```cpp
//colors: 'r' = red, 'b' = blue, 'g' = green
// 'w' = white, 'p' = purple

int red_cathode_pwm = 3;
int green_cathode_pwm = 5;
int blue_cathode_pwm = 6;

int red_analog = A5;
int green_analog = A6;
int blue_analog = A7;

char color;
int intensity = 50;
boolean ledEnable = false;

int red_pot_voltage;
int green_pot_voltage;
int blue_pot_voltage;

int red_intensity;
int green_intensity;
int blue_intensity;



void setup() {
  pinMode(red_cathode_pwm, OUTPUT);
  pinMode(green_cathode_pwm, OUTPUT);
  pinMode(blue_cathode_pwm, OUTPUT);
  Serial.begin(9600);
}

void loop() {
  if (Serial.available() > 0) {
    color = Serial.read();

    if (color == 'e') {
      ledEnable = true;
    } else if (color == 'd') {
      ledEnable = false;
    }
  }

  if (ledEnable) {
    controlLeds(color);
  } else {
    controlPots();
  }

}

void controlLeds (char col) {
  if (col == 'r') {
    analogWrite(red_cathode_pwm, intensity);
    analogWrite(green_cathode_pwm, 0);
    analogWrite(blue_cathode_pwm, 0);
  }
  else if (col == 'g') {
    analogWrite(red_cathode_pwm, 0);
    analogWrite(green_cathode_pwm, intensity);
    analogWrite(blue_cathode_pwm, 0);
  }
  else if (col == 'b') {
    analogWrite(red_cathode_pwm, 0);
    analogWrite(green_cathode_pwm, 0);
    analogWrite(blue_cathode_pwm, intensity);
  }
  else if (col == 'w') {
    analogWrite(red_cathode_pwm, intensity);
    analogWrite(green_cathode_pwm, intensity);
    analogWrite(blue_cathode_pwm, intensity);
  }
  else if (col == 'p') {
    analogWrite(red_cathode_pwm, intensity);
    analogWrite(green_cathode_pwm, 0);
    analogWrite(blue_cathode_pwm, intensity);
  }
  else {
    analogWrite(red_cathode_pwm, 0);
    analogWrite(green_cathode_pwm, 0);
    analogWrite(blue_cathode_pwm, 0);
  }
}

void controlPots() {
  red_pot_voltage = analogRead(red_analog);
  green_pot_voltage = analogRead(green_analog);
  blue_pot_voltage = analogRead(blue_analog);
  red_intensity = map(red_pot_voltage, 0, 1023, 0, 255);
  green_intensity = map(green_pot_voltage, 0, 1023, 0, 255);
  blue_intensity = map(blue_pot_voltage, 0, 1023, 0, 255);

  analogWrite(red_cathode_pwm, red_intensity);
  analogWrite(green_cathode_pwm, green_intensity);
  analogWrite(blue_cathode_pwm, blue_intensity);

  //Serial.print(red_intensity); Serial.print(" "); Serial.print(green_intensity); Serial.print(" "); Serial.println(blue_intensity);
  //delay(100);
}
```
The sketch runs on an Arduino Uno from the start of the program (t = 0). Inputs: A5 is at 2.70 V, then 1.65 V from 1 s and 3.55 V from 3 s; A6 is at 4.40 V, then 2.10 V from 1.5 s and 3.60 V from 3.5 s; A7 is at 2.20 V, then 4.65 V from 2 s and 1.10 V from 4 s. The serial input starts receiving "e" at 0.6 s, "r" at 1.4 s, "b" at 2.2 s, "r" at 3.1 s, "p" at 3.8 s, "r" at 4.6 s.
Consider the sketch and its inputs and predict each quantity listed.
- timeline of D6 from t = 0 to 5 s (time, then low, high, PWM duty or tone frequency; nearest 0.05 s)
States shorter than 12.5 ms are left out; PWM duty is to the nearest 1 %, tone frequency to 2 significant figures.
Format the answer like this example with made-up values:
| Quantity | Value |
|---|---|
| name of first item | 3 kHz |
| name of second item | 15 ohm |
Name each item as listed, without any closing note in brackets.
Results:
| Quantity | Value |
|---|---|
| timeline of D6 from t = 0 to 5 s | 0 s PWM 44 %; 0.6 s low; 2.2 s PWM 20 %; 3.1 s low; 3.8 s PWM 20 %; 4.6 s low |
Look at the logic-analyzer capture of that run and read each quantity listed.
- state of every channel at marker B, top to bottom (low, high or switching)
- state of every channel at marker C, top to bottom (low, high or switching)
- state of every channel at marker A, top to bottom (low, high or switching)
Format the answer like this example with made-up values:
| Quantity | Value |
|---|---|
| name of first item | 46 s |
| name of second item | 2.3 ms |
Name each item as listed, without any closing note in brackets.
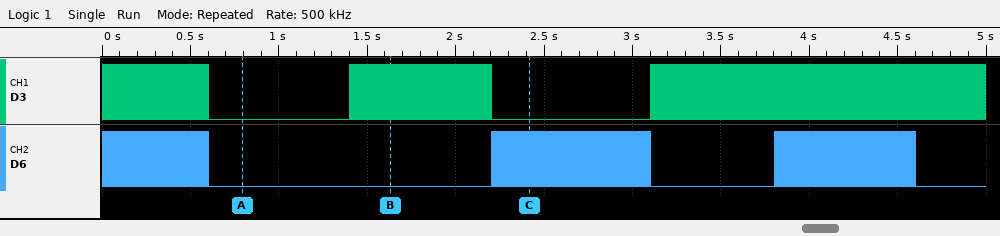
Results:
| Quantity | Value |
|---|---|
| state of every channel at marker B, top to bottom | D3 switching, D6 low |
| state of every channel at marker C, top to bottom | D3 low, D6 switching |
| state of every channel at marker A, top to bottom | D3 low, D6 low |
